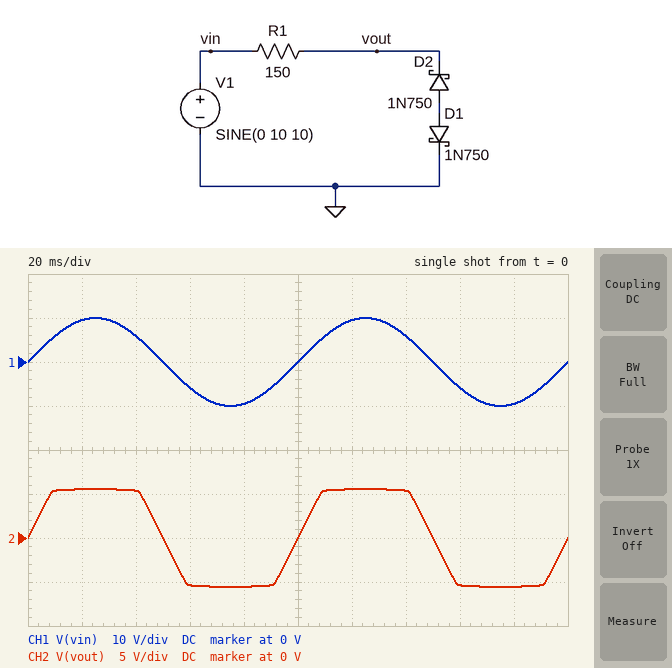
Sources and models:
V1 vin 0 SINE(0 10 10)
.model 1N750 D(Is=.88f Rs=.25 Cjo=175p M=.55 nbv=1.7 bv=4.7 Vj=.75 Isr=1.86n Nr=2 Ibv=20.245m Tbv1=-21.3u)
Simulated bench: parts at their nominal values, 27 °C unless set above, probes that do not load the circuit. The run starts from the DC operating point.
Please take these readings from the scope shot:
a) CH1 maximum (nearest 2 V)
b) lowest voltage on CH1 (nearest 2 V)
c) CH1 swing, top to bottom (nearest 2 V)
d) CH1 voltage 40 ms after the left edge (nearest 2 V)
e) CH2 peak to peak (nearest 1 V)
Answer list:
10 V
-10 V
20 V
6 V
11 V
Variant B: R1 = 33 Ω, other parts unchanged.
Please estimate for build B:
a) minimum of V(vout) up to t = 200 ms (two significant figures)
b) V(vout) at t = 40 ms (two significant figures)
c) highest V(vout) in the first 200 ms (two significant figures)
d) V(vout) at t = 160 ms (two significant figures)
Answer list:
-5.7 V
5.5 V
5.7 V
-5.5 V
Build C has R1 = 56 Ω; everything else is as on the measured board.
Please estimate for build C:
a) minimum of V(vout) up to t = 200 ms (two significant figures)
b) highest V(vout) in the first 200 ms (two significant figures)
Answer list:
-5.6 V
5.6 V
